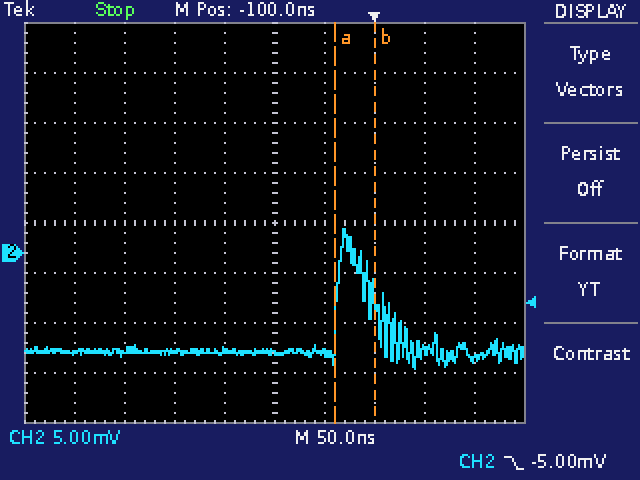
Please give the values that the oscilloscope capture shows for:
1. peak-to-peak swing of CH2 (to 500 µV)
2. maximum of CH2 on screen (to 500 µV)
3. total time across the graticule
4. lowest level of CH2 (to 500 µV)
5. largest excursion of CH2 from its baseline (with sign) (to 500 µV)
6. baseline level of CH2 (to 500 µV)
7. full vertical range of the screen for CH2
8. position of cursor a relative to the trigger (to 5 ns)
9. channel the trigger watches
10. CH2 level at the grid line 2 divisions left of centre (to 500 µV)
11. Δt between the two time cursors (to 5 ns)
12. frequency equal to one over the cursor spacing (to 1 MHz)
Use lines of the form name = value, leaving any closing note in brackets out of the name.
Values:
peak-to-peak swing of CH2 = 14.0 mV
maximum of CH2 on screen = 2.5 mV
total time across the graticule = 500 ns
lowest level of CH2 = -11.5 mV
largest excursion of CH2 from its baseline (with sign) = +12.5 mV
baseline level of CH2 = -10.0 mV
full vertical range of the screen for CH2 = 40 mV
position of cursor a relative to the trigger = -40 ns
channel the trigger watches = CH2
CH2 level at the grid line 2 divisions left of centre = -10.0 mV
Δt between the two time cursors = 40 ns
frequency equal to one over the cursor spacing = 25 MHz
